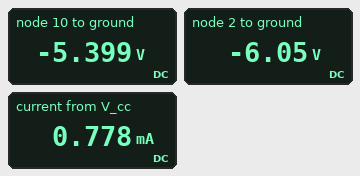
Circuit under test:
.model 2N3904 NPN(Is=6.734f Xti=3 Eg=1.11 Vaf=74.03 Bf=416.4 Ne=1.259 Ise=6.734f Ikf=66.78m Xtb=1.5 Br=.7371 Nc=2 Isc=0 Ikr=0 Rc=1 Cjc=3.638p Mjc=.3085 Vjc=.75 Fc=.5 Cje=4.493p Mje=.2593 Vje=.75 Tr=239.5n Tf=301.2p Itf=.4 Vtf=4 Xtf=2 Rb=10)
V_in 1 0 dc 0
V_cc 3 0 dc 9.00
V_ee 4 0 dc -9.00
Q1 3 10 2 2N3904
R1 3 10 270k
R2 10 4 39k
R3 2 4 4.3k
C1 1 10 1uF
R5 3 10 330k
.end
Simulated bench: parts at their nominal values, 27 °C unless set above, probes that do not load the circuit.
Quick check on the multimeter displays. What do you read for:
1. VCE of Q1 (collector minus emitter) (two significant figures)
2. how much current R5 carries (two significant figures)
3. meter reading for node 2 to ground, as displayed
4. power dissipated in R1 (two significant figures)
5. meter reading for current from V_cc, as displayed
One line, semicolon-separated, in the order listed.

15 V; 44 µA; -6.05 V; 770 µW; 0.778 mA
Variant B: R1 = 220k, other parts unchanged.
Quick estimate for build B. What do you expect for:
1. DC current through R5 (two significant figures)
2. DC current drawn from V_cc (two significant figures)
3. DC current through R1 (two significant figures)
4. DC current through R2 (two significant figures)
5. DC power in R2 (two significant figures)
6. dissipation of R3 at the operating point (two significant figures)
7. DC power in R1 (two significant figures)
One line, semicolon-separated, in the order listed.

43 µA; 870 µA; 64 µA; 100 µA; 400 µW; 2.5 mW; 900 µW
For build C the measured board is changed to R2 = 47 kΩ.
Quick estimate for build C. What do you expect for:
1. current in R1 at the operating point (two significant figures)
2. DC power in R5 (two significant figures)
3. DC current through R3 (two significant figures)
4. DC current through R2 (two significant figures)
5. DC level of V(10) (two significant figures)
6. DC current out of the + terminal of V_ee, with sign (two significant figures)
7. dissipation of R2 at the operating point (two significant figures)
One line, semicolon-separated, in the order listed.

51 µA; 580 µW; 810 µA; 88 µA; -4.9 V; -900 µA; 360 µW
